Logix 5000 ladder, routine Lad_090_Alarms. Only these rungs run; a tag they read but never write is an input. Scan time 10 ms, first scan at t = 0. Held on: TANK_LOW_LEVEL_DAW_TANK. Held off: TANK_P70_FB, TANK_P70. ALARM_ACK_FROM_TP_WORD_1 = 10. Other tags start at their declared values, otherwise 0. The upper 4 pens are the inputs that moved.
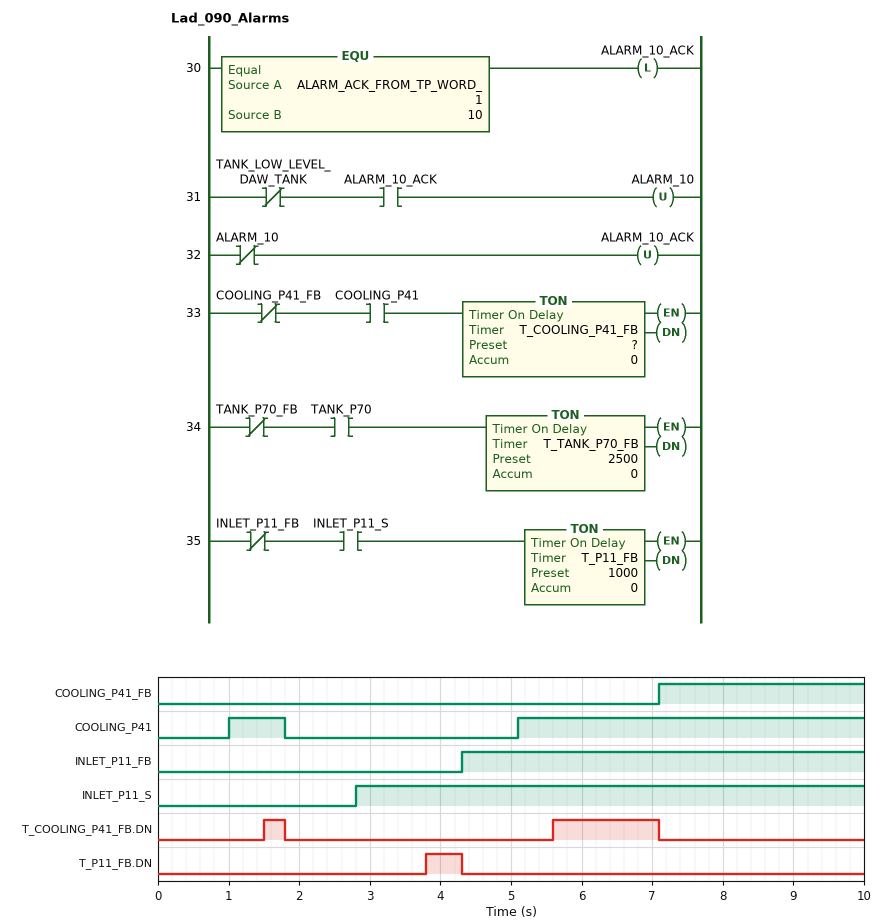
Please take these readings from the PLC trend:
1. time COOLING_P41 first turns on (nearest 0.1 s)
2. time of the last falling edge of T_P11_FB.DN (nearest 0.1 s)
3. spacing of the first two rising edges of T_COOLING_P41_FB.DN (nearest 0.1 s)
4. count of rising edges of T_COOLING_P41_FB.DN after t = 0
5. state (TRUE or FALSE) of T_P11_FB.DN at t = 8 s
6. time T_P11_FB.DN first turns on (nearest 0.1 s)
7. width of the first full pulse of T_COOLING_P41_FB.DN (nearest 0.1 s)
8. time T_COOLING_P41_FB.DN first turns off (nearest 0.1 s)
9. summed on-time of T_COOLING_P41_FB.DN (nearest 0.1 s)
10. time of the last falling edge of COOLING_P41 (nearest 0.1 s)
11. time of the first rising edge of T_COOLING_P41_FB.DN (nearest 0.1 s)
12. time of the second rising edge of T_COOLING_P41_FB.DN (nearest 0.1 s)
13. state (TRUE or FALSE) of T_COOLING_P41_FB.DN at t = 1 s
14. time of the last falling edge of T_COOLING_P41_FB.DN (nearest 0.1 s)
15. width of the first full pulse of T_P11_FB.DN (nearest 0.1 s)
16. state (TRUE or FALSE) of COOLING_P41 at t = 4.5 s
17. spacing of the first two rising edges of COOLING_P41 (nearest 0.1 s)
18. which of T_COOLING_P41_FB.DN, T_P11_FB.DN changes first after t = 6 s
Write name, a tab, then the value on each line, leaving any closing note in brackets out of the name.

time COOLING_P41 first turns on	1.0 s
time of the last falling edge of T_P11_FB.DN	4.3 s
spacing of the first two rising edges of T_COOLING_P41_FB.DN	4.1 s
count of rising edges of T_COOLING_P41_FB.DN after t = 0	2
state (TRUE or FALSE) of T_P11_FB.DN at t = 8 s	FALSE
time T_P11_FB.DN first turns on	3.8 s
width of the first full pulse of T_COOLING_P41_FB.DN	0.3 s
time T_COOLING_P41_FB.DN first turns off	1.8 s
summed on-time of T_COOLING_P41_FB.DN	1.8 s
time of the last falling edge of COOLING_P41	1.8 s
time of the first rising edge of T_COOLING_P41_FB.DN	1.5 s
time of the second rising edge of T_COOLING_P41_FB.DN	5.6 s
state (TRUE or FALSE) of T_COOLING_P41_FB.DN at t = 1 s	FALSE
time of the last falling edge of T_COOLING_P41_FB.DN	7.1 s
width of the first full pulse of T_P11_FB.DN	0.5 s
state (TRUE or FALSE) of COOLING_P41 at t = 4.5 s	FALSE
spacing of the first two rising edges of COOLING_P41	4.1 s
which of T_COOLING_P41_FB.DN, T_P11_FB.DN changes first after t = 6 s	T_COOLING_P41_FB.DN
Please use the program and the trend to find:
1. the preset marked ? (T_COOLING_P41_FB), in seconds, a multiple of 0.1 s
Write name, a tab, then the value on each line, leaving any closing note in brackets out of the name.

the preset marked ? (T_COOLING_P41_FB), in seconds, a multiple of 0.1 s	0.5 s
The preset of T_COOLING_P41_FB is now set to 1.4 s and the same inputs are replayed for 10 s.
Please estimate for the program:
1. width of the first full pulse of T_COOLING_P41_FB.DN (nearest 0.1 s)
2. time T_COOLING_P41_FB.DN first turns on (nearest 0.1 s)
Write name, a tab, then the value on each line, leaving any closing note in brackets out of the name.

width of the first full pulse of T_COOLING_P41_FB.DN	0.6 s
time T_COOLING_P41_FB.DN first turns on	6.5 s
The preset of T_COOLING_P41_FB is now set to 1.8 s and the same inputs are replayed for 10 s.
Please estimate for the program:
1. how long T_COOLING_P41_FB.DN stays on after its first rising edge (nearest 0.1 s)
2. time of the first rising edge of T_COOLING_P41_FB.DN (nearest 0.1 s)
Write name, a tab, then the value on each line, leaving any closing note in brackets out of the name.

how long T_COOLING_P41_FB.DN stays on after its first rising edge	0.2 s
time of the first rising edge of T_COOLING_P41_FB.DN	6.9 s
